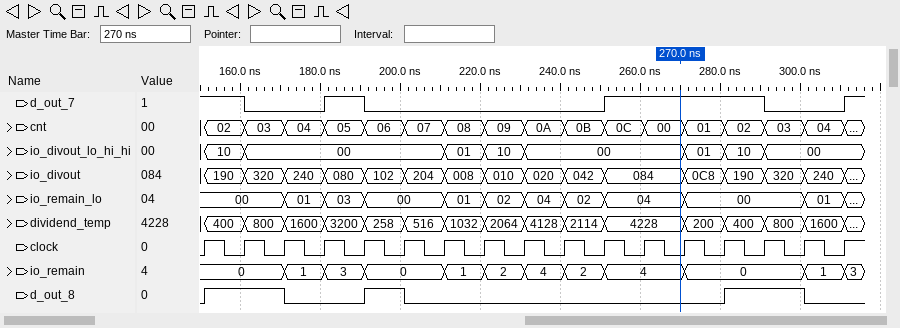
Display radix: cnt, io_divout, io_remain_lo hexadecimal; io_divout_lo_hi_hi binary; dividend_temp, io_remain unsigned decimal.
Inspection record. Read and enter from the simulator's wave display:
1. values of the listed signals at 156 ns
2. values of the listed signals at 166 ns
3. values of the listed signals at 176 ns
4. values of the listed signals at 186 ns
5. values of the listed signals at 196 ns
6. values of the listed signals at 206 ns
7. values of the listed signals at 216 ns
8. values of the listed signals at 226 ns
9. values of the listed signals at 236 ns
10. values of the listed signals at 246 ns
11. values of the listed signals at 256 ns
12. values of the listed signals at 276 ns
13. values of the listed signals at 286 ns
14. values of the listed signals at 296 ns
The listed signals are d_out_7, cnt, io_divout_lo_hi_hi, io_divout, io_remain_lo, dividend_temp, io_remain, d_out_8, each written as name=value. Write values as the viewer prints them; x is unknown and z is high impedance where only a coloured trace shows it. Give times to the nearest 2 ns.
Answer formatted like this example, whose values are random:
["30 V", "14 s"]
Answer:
["d_out_7=1, cnt=02, io_divout_lo_hi_hi=10, io_divout=190, io_remain_lo=00, dividend_temp=400, io_remain=0, d_out_8=1", "d_out_7=0, cnt=03, io_divout_lo_hi_hi=00, io_divout=320, io_remain_lo=00, dividend_temp=800, io_remain=0, d_out_8=1", "d_out_7=0, cnt=04, io_divout_lo_hi_hi=00, io_divout=240, io_remain_lo=01, dividend_temp=1600, io_remain=1, d_out_8=0", "d_out_7=1, cnt=05, io_divout_lo_hi_hi=00, io_divout=080, io_remain_lo=03, dividend_temp=3200, io_remain=3, d_out_8=0", "d_out_7=0, cnt=06, io_divout_lo_hi_hi=00, io_divout=102, io_remain_lo=00, dividend_temp=258, io_remain=0, d_out_8=1", "d_out_7=0, cnt=07, io_divout_lo_hi_hi=00, io_divout=204, io_remain_lo=00, dividend_temp=516, io_remain=0, d_out_8=0", "d_out_7=0, cnt=08, io_divout_lo_hi_hi=01, io_divout=008, io_remain_lo=01, dividend_temp=1032, io_remain=1, d_out_8=0", "d_out_7=0, cnt=09, io_divout_lo_hi_hi=10, io_divout=010, io_remain_lo=02, dividend_temp=2064, io_remain=2, d_out_8=0", "d_out_7=0, cnt=0A, io_divout_lo_hi_hi=00, io_divout=020, io_remain_lo=04, dividend_temp=4128, io_remain=4, d_out_8=0", "d_out_7=0, cnt=0B, io_divout_lo_hi_hi=00, io_divout=042, io_remain_lo=02, dividend_temp=2114, io_remain=2, d_out_8=0", "d_out_7=1, cnt=0C, io_divout_lo_hi_hi=00, io_divout=084, io_remain_lo=04, dividend_temp=4228, io_remain=4, d_out_8=0", "d_out_7=1, cnt=01, io_divout_lo_hi_hi=01, io_divout=0C8, io_remain_lo=00, dividend_temp=200, io_remain=0, d_out_8=0", "d_out_7=1, cnt=02, io_divout_lo_hi_hi=10, io_divout=190, io_remain_lo=00, dividend_temp=400, io_remain=0, d_out_8=1", "d_out_7=0, cnt=03, io_divout_lo_hi_hi=00, io_divout=320, io_remain_lo=00, dividend_temp=800, io_remain=0, d_out_8=1"]
